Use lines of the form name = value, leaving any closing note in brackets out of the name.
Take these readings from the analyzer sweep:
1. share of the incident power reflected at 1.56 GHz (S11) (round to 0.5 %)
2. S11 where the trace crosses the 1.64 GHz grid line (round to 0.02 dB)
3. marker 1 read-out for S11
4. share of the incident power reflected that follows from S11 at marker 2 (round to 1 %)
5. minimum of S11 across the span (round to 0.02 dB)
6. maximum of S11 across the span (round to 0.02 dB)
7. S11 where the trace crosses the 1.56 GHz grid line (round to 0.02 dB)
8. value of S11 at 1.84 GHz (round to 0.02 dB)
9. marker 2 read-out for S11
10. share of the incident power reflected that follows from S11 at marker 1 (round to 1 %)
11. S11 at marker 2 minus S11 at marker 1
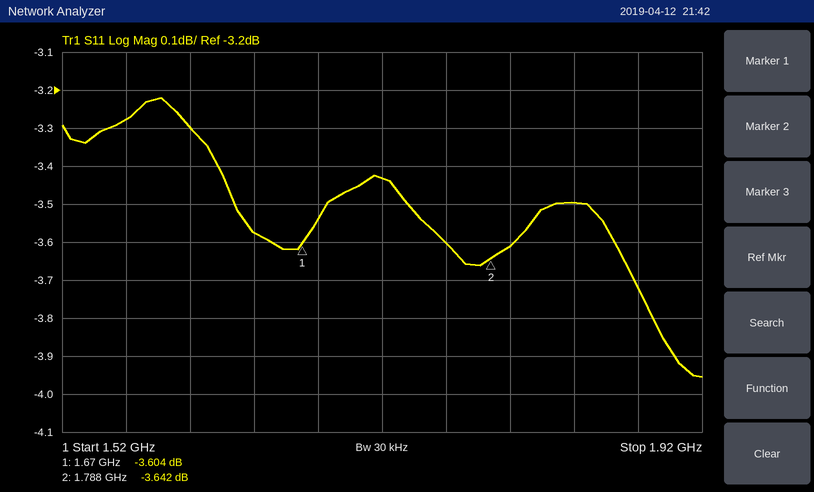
share of the incident power reflected at 1.56 GHz (S11) = 47.0 %
S11 where the trace crosses the 1.64 GHz grid line = -3.58 dB
marker 1 read-out for S11 = -3.604 dB
share of the incident power reflected that follows from S11 at marker 2 = 43 %
minimum of S11 across the span = -3.96 dB
maximum of S11 across the span = -3.22 dB
S11 where the trace crosses the 1.56 GHz grid line = -3.28 dB
value of S11 at 1.84 GHz = -3.50 dB
marker 2 read-out for S11 = -3.642 dB
share of the incident power reflected that follows from S11 at marker 1 = 44 %
S11 at marker 2 minus S11 at marker 1 = -0.038 dB
